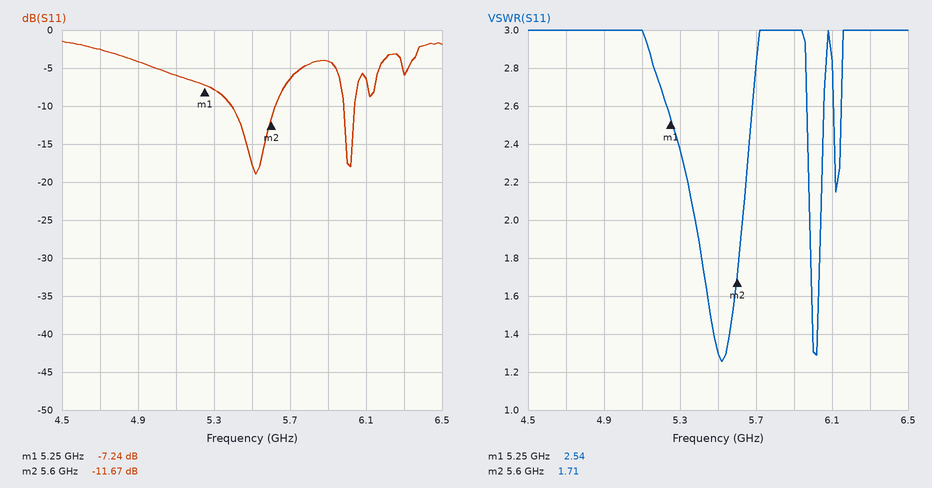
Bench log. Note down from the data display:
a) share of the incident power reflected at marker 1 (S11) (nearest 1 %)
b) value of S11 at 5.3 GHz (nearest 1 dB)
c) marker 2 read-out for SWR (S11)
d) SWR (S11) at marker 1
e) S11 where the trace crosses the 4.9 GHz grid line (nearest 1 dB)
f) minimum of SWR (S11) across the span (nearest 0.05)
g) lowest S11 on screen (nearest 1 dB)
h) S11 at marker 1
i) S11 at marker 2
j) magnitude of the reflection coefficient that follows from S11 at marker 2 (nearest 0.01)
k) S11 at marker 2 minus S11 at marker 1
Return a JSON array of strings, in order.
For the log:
["19 %", "-8 dB", "1.71", "2.54", "-4 dB", "1.25", "-19 dB", "-7.24 dB", "-11.67 dB", "0.26", "-4.43 dB"]
